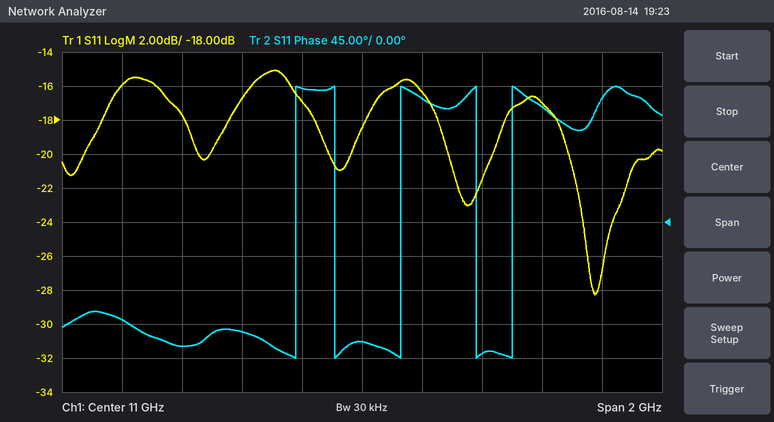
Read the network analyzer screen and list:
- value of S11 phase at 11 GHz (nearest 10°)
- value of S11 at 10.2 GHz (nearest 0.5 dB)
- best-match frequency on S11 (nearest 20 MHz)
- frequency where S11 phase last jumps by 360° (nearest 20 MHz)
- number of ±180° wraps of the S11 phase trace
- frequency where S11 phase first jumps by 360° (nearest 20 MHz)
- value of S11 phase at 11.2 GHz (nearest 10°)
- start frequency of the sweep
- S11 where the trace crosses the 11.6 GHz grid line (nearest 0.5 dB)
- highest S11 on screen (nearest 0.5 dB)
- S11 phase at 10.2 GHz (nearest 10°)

-160°
-16.0 dB
11.78 GHz
11.50 GHz
5
10.78 GHz
160°
10 GHz
-17.0 dB
-15.0 dB
-130°
